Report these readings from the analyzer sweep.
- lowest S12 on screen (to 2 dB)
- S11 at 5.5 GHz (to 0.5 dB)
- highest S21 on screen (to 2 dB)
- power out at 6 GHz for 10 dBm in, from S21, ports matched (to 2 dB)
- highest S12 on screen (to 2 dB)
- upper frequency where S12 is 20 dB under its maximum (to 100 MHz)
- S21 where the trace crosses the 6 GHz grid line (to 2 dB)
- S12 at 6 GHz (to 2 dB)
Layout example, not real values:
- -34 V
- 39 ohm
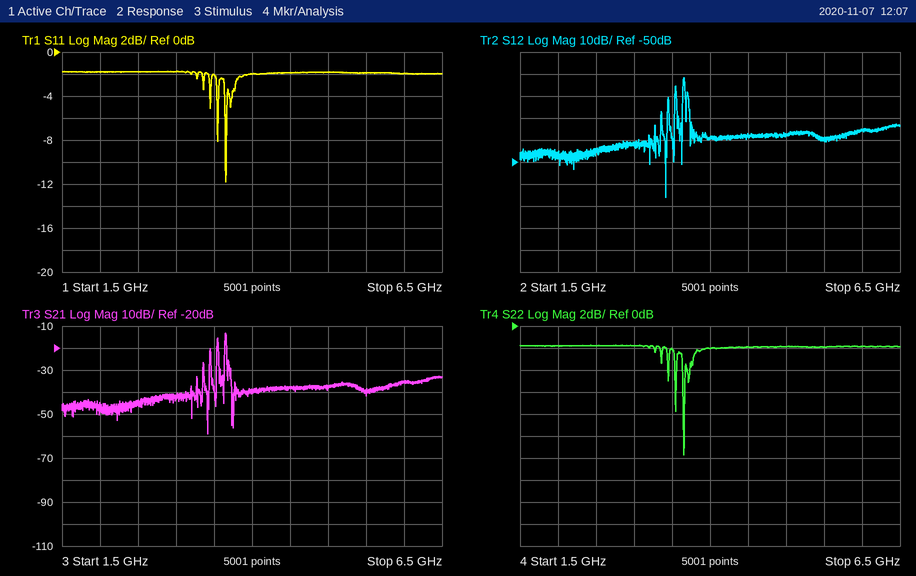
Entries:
- -66 dB
- -2.0 dB
- -14 dB
- -26 dBm
- -12 dB
- 3.7 GHz
- -36 dB
- -36 dB
